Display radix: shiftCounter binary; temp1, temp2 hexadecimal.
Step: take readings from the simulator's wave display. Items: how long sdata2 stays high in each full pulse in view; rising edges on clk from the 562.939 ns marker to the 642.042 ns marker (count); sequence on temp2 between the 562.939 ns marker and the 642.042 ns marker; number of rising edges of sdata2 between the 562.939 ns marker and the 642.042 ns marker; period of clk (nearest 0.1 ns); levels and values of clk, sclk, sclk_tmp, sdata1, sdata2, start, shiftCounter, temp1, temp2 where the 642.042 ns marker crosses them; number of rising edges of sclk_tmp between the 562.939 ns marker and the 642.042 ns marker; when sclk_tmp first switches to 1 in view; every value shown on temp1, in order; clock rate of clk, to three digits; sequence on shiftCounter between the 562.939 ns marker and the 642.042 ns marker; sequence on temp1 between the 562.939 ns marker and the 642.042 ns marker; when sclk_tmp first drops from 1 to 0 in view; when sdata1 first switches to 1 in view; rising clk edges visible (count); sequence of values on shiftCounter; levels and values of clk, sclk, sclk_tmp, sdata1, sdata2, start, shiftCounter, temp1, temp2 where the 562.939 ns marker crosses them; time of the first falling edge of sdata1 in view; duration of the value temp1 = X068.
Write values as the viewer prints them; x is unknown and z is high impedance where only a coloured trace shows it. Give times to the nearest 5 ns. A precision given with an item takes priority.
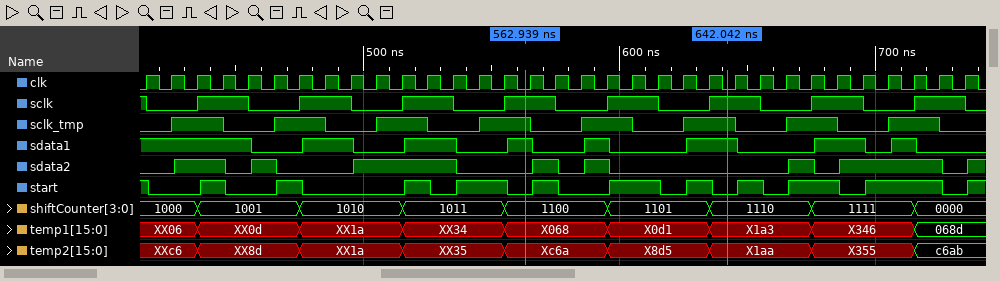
20 ns, 10 ns, 40 ns, 10 ns, 10 ns, 10 ns, 40 ns
8
Xc6a, X8d5, X1aa
2
10 ns
clk=0, sclk=1, sclk_tmp=1, sdata1=1, sdata2=0, start=0, shiftCounter=1110, temp1=X1a3, temp2=X1aa
2
425 ns
XX06, XX0d, XX1a, XX34, X068, X0d1, X1a3, X346, 068d
100 MHz
1100, 1101, 1110
X068, X0d1, X1a3
445 ns
475 ns
33
1000, 1001, 1010, 1011, 1100, 1101, 1110, 1111, 0000
clk=0, sclk=1, sclk_tmp=1, sdata1=1, sdata2=0, start=0, shiftCounter=1100, temp1=X068, temp2=Xc6a
455 ns
40 ns
